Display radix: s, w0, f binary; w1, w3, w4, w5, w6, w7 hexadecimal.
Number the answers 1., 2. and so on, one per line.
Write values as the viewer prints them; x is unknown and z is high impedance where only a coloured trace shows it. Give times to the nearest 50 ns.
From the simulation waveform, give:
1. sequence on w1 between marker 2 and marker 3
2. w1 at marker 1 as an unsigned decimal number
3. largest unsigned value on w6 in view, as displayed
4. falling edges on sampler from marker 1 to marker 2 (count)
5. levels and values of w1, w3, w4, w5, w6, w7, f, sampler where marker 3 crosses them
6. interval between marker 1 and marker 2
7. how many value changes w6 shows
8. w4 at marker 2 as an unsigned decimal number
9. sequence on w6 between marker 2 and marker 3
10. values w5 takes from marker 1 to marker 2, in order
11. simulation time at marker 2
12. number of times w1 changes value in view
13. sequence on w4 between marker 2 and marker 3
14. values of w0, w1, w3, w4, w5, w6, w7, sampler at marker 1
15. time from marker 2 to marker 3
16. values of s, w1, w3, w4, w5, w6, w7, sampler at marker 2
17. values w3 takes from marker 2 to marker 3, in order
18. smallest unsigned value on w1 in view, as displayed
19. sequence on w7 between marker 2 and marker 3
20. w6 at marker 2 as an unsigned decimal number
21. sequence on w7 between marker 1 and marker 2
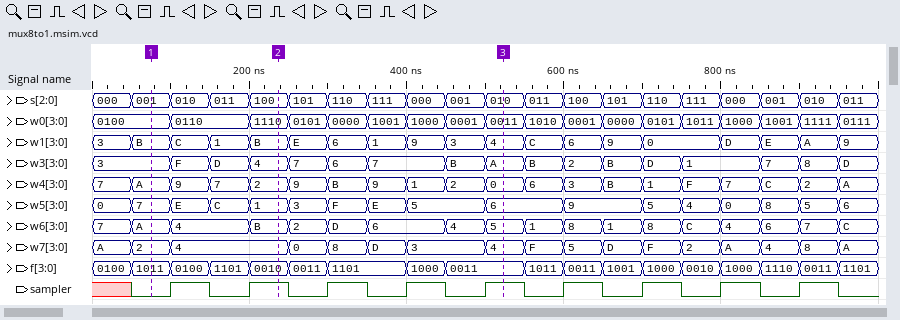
1. B, E, 6, 1, 9, 3, 4
2. 11
3. D
4. 1
5. w1=4, w3=A, w4=0, w5=6, w6=5, w7=4, f=0011, sampler=1
6. 150 ns
7. 17
8. 2
9. B, 2, D, 6, 4, 5
10. 7, E, C, 1
11. 250 ns
12. 18
13. 2, 9, B, 9, 1, 2, 0
14. w0=0100, w1=B, w3=3, w4=A, w5=7, w6=A, w7=2, sampler=0
15. 300 ns
16. s=100, w1=B, w3=4, w4=2, w5=1, w6=B, w7=4, sampler=1
17. 4, 7, 6, 7, B, A
18. 0
19. 4, 0, 8, D, 3, 4
20. 11
21. 2, 4
